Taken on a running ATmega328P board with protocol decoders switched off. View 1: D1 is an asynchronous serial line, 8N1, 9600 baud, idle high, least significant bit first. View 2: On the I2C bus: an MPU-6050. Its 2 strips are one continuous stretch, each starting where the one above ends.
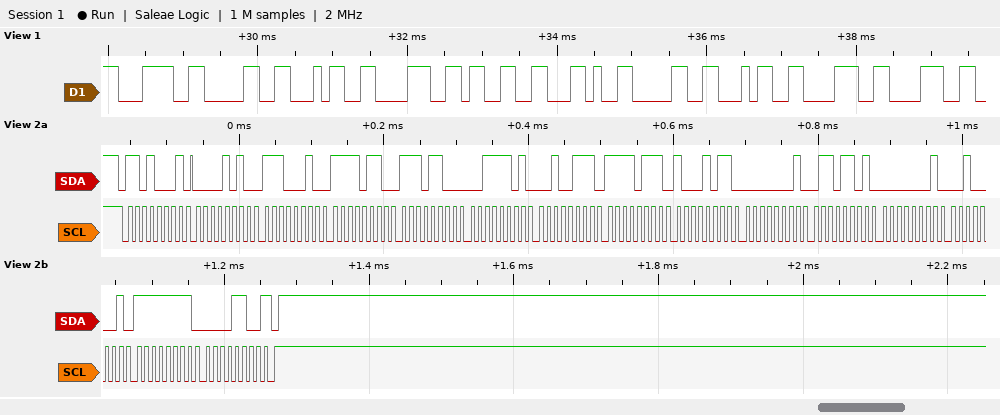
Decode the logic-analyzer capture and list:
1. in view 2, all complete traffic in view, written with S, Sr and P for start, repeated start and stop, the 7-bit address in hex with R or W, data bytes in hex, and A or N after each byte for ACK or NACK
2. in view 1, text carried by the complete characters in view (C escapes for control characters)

S 68R A 0A A E2 A F6 A EC A 3D A 27 A F7 A 8B A 01 A 6D A 01 A 21 A FF A 0C N P
"<0483,0488"
